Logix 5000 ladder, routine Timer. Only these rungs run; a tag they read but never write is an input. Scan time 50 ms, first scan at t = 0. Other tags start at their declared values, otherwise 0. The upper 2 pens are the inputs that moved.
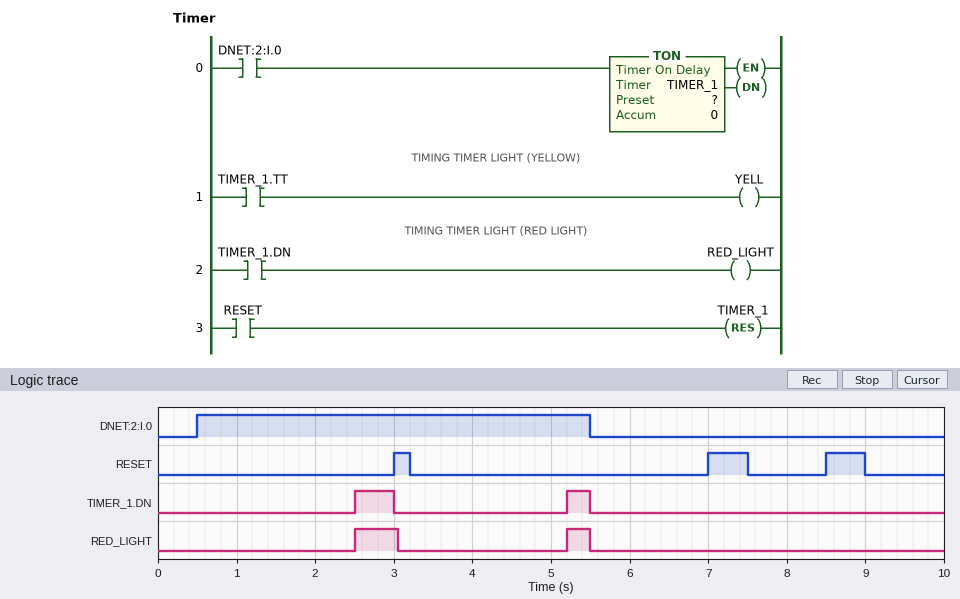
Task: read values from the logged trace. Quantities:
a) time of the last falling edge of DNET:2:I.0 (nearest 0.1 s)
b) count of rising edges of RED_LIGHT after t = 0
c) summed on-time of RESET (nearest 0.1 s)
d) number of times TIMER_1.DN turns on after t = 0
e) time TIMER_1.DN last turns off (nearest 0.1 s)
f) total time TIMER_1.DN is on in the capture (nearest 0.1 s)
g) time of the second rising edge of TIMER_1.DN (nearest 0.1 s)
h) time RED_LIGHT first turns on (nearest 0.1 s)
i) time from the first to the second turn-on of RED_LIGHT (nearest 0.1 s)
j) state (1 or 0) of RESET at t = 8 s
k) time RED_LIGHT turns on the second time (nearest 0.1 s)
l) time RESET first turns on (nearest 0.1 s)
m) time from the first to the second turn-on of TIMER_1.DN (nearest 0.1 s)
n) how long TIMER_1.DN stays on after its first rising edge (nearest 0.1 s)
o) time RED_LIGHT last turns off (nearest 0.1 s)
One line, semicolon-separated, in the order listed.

5.5 s; 2; 1.2 s; 2; 5.5 s; 0.8 s; 5.2 s; 2.5 s; 2.7 s; 0; 5.2 s; 3.0 s; 2.7 s; 0.5 s; 5.5 s
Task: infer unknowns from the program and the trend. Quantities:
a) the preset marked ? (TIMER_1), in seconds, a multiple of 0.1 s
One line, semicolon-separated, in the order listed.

2.0 s
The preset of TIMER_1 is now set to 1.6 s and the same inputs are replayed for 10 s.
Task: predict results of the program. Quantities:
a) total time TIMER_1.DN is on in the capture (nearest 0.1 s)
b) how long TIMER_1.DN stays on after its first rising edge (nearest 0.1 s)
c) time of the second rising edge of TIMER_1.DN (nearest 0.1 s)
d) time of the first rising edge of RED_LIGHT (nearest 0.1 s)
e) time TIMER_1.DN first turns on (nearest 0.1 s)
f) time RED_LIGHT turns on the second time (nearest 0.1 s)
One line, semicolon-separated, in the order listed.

1.6 s; 0.9 s; 4.8 s; 2.1 s; 2.1 s; 4.8 s
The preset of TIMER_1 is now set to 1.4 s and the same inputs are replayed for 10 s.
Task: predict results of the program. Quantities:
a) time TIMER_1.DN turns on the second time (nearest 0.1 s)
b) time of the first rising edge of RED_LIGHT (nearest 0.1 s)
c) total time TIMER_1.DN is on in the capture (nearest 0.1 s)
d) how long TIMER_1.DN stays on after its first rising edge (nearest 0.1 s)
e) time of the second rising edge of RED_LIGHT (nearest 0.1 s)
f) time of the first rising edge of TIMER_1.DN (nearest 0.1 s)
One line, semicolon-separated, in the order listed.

4.6 s; 1.9 s; 2.0 s; 1.1 s; 4.6 s; 1.9 s
